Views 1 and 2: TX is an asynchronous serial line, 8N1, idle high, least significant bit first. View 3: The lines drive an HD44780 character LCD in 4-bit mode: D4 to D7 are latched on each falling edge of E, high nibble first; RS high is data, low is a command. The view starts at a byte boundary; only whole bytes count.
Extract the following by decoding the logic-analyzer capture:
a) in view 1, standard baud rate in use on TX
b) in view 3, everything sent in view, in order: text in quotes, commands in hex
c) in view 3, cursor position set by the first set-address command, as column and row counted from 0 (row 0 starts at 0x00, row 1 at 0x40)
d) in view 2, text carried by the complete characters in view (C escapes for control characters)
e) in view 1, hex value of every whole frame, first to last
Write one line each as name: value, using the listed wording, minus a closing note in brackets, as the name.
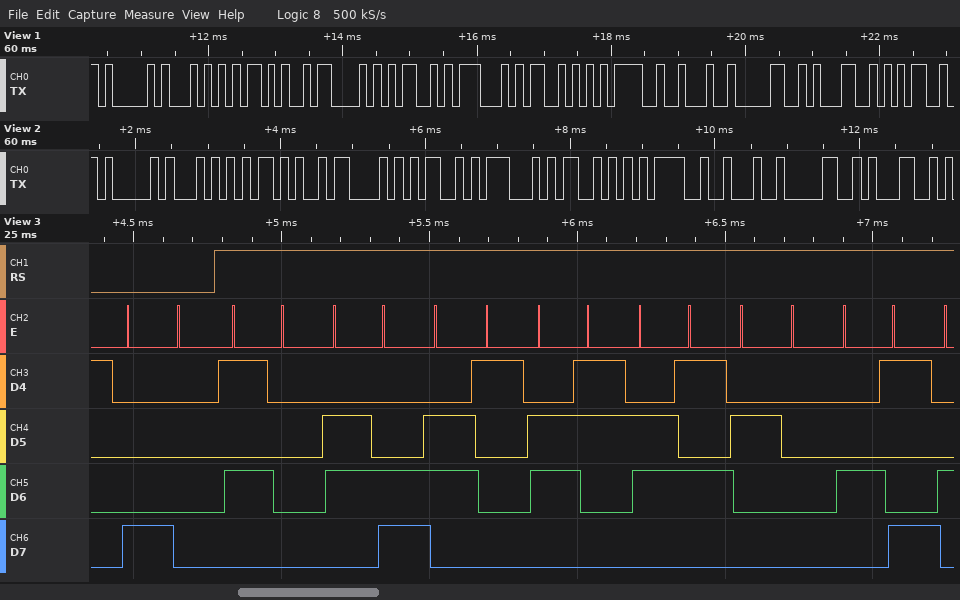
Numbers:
in view 1, standard baud rate in use on TX: 9600 baud
in view 3, everything sent in view, in order: text in quotes, commands in hex: 0x80 "Place I"
in view 3, cursor position set by the first set-address command, as column and row counted from 0: column 0, row 0
in view 2, text carried by the complete characters in view: "AT+CMGS=\"01"
in view 1, hex value of every whole frame, first to last: 41 54 2B 43 4D 47 53 3D 22 30 31 35
